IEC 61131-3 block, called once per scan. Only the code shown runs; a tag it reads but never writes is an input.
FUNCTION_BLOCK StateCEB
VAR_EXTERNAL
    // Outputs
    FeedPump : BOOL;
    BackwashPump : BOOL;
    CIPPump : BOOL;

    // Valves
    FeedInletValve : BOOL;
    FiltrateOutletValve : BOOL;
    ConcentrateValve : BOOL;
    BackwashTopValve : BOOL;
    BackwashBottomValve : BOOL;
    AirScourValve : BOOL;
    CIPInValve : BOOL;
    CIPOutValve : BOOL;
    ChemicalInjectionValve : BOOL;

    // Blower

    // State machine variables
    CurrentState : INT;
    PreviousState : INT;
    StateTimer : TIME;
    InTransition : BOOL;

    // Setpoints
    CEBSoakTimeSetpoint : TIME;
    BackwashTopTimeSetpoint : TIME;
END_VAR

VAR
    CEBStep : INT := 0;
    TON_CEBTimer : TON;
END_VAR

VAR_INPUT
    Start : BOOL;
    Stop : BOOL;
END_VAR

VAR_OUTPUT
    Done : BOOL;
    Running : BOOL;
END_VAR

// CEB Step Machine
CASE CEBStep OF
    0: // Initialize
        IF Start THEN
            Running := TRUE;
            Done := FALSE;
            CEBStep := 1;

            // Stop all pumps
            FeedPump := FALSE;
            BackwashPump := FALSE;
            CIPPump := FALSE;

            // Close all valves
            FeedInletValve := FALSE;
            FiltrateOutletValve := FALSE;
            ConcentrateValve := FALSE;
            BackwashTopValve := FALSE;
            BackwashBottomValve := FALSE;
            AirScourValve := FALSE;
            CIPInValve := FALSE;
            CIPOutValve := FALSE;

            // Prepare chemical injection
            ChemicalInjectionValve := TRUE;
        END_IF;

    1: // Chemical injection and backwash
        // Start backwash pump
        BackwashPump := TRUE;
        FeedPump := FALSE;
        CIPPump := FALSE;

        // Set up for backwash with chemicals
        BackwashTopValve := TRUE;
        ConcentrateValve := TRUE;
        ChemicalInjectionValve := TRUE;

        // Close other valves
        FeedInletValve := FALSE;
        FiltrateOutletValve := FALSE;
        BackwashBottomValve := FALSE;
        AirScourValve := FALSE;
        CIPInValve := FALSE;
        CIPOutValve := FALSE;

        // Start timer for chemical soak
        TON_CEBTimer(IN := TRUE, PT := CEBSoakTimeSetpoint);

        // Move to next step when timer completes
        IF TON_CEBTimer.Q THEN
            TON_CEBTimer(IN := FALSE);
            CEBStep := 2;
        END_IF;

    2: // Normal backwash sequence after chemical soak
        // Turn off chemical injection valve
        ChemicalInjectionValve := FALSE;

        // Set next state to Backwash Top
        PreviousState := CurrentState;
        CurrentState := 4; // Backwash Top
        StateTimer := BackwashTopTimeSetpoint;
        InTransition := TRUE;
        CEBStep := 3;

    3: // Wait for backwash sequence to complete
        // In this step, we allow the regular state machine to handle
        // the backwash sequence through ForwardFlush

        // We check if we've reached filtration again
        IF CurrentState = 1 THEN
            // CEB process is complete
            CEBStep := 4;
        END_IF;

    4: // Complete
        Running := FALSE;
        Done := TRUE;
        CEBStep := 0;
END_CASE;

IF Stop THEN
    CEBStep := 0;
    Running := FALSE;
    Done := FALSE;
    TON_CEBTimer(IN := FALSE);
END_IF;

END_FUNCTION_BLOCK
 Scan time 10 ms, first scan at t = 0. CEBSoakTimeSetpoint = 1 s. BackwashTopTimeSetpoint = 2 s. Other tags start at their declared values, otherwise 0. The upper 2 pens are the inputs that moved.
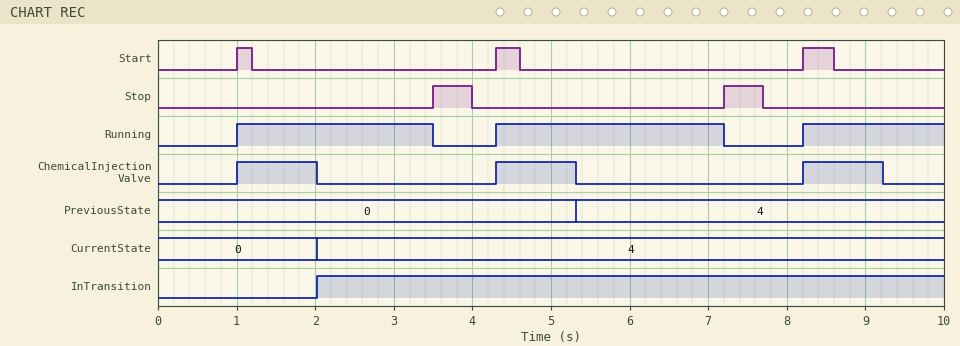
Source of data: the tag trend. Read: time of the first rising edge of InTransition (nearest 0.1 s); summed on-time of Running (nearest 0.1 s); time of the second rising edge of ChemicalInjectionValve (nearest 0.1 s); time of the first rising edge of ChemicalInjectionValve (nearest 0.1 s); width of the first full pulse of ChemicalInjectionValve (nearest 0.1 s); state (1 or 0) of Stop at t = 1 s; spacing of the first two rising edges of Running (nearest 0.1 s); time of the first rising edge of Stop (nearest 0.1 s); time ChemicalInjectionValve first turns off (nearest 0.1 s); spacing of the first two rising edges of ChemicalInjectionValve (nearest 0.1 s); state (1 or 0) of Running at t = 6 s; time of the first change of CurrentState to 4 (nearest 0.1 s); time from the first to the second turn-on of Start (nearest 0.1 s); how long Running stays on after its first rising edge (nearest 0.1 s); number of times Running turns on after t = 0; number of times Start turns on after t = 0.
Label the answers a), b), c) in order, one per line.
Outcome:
a) 2.0 s
b) 7.2 s
c) 4.3 s
d) 1.0 s
e) 1.0 s
f) 0
g) 3.3 s
h) 3.5 s
i) 2.0 s
j) 3.3 s
k) 1
l) 2.0 s
m) 3.3 s
n) 2.5 s
o) 3
p) 3
